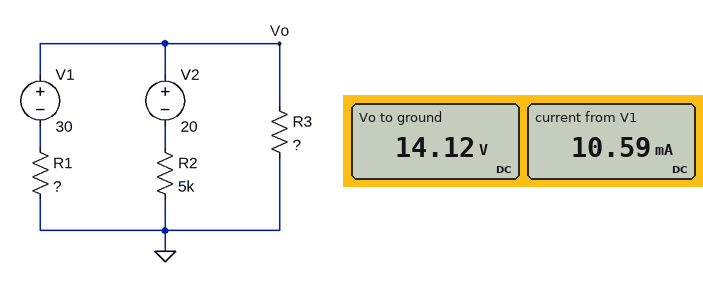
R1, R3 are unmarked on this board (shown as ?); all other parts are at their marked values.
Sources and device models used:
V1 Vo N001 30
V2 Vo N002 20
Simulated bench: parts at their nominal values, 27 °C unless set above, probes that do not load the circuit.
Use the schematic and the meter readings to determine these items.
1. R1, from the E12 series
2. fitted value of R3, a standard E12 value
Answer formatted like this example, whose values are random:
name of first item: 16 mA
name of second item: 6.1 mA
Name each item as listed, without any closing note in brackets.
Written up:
R1, from the E12 series: 1.5 kΩ
fitted value of R3, a standard E12 value: 1.2 kΩ
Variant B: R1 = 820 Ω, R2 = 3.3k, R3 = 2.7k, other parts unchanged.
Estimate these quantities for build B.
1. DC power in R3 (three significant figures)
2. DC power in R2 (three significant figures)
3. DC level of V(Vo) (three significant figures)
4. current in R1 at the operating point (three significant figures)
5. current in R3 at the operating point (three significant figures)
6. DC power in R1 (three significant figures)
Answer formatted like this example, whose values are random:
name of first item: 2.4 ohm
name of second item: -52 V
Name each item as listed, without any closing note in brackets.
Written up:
DC power in R3: 188 mW
DC power in R2: 1.94 mW
DC level of V(Vo): 22.5 V
current in R1 at the operating point: 9.11 mA
current in R3 at the operating point: 8.34 mA
DC power in R1: 68.1 mW
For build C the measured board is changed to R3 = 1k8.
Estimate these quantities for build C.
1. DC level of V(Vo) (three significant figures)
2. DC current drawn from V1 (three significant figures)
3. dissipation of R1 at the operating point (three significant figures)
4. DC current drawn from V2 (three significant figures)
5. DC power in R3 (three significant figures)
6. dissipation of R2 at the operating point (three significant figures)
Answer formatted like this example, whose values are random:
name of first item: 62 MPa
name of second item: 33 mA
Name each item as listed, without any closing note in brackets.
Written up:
DC level of V(Vo): 16.9 V
DC current drawn from V1: 8.75 mA
dissipation of R1 at the operating point: 115 mW
DC current drawn from V2: 625 µA
DC power in R3: 158 mW
dissipation of R2 at the operating point: 1.95 mW
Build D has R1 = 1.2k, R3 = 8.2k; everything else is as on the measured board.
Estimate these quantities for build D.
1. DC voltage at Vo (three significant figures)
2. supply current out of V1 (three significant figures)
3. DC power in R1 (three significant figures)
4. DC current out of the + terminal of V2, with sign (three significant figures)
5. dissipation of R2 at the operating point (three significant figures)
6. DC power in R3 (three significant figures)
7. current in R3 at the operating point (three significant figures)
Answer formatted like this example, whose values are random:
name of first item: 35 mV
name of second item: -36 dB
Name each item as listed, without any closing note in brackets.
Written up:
DC voltage at Vo: 25.1 V
supply current out of V1: 4.08 mA
DC power in R1: 20.0 mW
DC current out of the + terminal of V2, with sign: -1.02 mA
dissipation of R2 at the operating point: 5.21 mW
DC power in R3: 76.8 mW
current in R3 at the operating point: 3.06 mA
